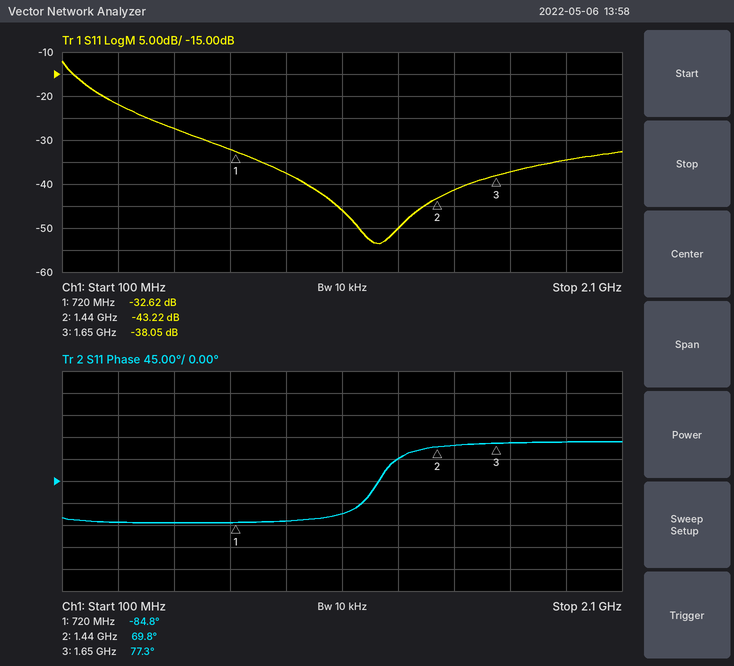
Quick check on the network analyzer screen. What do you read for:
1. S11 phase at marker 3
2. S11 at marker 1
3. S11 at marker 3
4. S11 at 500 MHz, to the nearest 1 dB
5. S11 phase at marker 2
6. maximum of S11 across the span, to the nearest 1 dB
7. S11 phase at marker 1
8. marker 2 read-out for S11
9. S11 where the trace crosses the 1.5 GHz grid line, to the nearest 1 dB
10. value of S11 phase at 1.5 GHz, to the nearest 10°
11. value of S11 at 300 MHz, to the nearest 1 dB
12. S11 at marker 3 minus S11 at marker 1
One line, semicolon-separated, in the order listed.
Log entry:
77.3°; -32.62 dB; -38.05 dB; -27 dB; 69.8°; -12 dB; -84.8°; -43.22 dB; -41 dB; 70°; -22 dB; -5.43 dB
